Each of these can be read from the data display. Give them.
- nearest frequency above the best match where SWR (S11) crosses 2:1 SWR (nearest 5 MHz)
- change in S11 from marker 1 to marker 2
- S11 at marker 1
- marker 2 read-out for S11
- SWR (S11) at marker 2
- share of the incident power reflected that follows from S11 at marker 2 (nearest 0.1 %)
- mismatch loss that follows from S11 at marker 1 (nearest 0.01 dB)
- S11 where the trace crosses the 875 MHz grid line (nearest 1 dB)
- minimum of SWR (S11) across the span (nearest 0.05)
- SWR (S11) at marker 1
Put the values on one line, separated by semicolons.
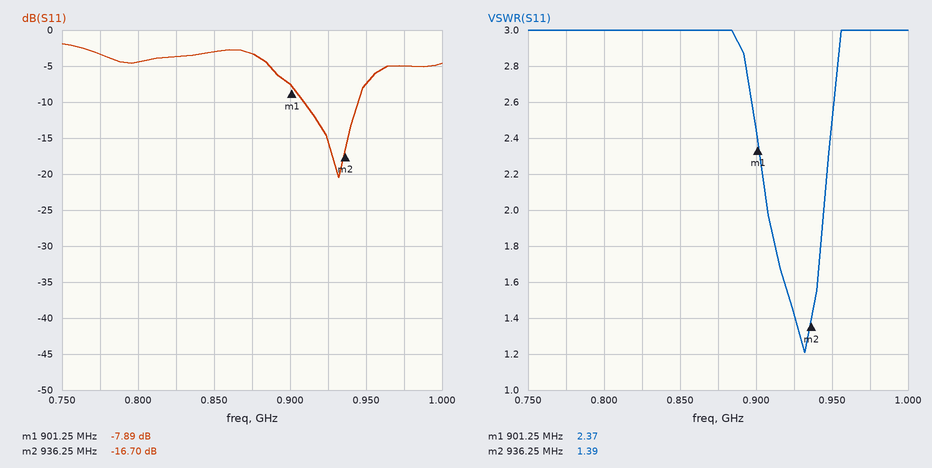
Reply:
945 MHz; -8.81 dB; -7.89 dB; -16.70 dB; 1.39; 2.1 %; 0.77 dB; -3 dB; 1.20; 2.37
